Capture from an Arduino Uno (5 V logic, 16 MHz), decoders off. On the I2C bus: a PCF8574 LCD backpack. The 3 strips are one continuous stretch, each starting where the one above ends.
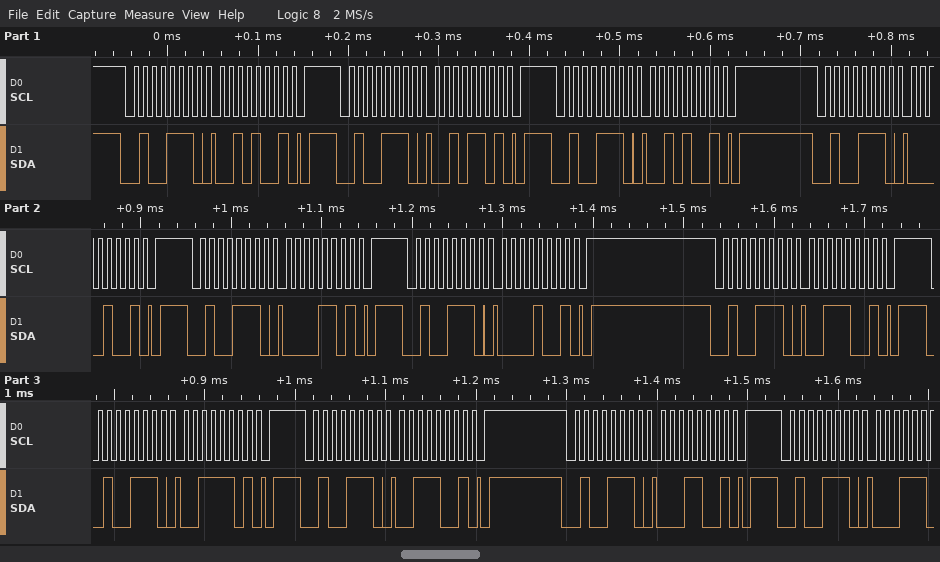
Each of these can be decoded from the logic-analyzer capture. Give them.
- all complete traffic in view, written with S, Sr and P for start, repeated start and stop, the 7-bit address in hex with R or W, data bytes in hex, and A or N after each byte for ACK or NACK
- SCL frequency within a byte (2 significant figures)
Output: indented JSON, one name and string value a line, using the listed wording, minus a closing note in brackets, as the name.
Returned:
{
  "all complete traffic in view, written with S, Sr and P for start, repeated start and stop, the 7-bit address in hex with R or W, data bytes in hex, and A or N after each byte for ACK or NACK": "S 27W A 29 A P S 27W A 2D A P S 27W A 29 A P S 27W A 09 A P S 27W A 0D A P S 27W A 09 A P S 27W A 39 A P S 27W A 3D A P S 27W A 39 A P S 27W A 19 A P S 27W A",
  "SCL frequency within a byte": "100 kHz"
}
